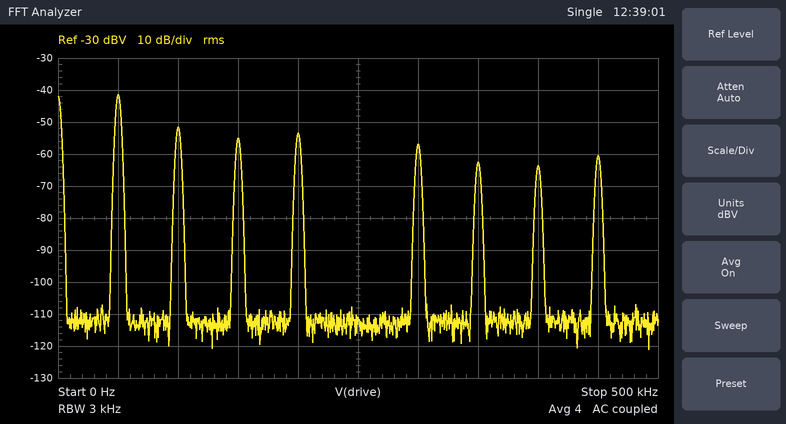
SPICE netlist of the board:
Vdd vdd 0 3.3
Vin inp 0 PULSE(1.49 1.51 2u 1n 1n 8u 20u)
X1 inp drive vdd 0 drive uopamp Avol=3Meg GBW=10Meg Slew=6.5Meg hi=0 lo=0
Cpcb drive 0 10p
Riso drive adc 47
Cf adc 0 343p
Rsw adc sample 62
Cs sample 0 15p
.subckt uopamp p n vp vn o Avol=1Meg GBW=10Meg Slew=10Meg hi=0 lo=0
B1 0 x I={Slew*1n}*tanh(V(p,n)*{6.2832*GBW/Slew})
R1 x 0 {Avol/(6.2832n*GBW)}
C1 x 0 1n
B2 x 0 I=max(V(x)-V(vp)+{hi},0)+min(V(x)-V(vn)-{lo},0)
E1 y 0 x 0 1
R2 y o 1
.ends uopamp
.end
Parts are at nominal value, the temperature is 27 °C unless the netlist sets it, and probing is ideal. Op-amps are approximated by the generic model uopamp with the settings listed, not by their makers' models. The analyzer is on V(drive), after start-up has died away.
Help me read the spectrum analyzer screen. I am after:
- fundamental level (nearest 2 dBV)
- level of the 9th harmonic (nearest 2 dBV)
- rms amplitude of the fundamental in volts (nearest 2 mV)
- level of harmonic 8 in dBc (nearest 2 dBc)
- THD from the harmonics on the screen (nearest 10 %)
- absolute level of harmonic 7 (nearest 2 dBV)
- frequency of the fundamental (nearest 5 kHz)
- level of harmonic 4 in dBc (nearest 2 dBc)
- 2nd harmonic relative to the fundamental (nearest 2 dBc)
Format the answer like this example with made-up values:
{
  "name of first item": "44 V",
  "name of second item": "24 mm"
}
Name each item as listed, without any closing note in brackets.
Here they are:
{
  "fundamental level": "-42 dBV",
  "level of the 9th harmonic": "-60 dBV",
  "rms amplitude of the fundamental in volts": "8 mV",
  "level of harmonic 8 in dBc": "-22 dBc",
  "THD from the harmonics on the screen": "50 %",
  "absolute level of harmonic 7": "-62 dBV",
  "frequency of the fundamental": "50 kHz",
  "level of harmonic 4 in dBc": "-12 dBc",
  "2nd harmonic relative to the fundamental": "-10 dBc"
}
